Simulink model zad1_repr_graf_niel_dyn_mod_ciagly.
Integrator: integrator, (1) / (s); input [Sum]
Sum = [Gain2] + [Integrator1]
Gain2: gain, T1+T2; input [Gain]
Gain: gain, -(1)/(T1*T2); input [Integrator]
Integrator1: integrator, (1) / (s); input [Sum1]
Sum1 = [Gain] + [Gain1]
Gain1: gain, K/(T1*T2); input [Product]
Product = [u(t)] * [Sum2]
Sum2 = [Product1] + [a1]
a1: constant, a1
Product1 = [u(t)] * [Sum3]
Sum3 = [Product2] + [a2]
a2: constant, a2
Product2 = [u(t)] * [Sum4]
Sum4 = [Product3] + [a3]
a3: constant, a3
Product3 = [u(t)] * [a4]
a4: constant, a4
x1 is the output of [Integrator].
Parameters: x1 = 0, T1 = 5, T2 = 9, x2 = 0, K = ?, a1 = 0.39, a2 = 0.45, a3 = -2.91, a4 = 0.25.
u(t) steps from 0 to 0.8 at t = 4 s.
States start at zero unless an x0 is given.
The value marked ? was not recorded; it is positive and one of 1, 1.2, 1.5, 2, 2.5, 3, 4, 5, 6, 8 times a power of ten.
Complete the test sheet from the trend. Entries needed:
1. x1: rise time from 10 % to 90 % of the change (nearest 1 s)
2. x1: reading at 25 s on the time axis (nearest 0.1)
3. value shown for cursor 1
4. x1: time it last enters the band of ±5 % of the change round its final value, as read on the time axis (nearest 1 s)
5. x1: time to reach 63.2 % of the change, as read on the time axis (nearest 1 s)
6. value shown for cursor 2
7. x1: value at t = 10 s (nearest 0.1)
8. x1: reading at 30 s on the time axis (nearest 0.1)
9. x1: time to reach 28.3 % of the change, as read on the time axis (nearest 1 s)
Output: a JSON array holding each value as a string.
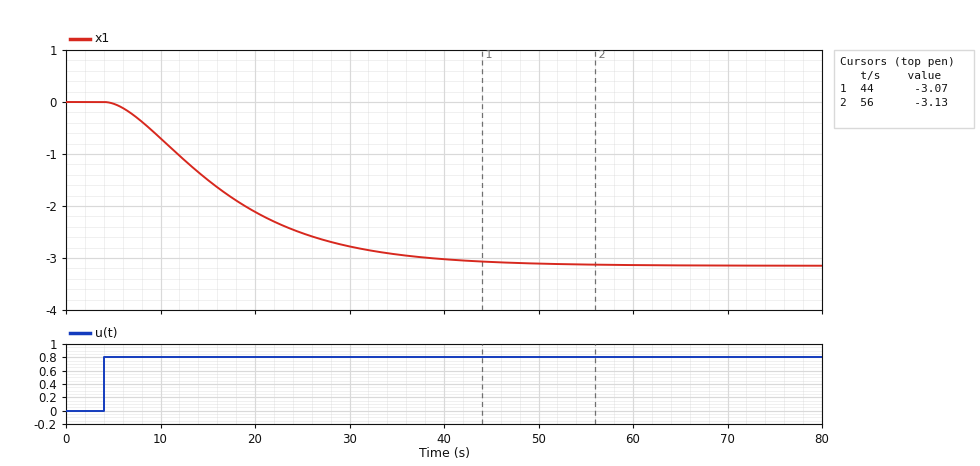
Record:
["24 s", "-2.5", "-3.07", "38 s", "19 s", "-3.13", "-0.7", "-2.8", "11 s"]
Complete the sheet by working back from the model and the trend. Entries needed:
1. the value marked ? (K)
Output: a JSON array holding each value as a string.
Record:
["4"]
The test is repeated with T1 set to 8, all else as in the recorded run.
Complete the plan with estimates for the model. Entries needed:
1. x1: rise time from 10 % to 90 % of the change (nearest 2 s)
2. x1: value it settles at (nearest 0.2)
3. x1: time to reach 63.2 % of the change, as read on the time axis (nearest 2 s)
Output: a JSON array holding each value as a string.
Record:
["28 s", "-3.2", "22 s"]
